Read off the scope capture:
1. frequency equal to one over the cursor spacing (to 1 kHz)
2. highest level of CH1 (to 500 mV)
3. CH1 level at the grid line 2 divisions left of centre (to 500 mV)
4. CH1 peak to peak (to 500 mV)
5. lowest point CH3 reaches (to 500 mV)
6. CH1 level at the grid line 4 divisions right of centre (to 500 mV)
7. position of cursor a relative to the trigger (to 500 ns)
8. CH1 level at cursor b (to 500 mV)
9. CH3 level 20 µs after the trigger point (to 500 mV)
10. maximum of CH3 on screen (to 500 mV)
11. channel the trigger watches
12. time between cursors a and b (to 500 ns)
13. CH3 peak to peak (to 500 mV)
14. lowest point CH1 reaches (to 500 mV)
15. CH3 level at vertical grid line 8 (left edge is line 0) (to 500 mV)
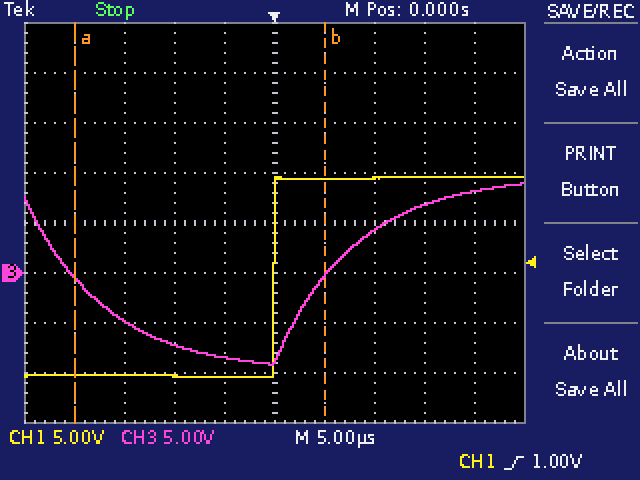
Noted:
40 kHz
9.5 V
-10.5 V
20.0 V
-9.0 V
9.5 V
-20.0 µs
9.5 V
8.0 V
9.0 V
CH1
25.0 µs
18.0 V
-10.5 V
7.0 V
